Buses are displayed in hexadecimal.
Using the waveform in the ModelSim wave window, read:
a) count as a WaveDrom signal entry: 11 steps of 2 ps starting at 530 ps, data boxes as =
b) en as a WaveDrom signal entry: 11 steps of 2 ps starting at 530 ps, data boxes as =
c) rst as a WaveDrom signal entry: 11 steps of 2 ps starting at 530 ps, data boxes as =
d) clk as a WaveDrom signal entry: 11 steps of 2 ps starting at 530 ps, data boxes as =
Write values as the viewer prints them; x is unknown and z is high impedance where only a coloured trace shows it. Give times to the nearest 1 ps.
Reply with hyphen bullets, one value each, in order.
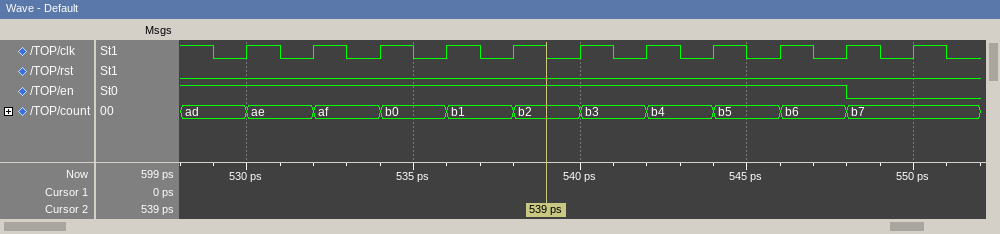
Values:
- {name: 'count', wave: '==========.', data: 'ae af b0 b1 b2 b3 b4 b5 b6 b7'}
- {name: 'en', wave: '1........0.'}
- {name: 'rst', wave: '0..........'}
- {name: 'clk', wave: 'p..........'}
